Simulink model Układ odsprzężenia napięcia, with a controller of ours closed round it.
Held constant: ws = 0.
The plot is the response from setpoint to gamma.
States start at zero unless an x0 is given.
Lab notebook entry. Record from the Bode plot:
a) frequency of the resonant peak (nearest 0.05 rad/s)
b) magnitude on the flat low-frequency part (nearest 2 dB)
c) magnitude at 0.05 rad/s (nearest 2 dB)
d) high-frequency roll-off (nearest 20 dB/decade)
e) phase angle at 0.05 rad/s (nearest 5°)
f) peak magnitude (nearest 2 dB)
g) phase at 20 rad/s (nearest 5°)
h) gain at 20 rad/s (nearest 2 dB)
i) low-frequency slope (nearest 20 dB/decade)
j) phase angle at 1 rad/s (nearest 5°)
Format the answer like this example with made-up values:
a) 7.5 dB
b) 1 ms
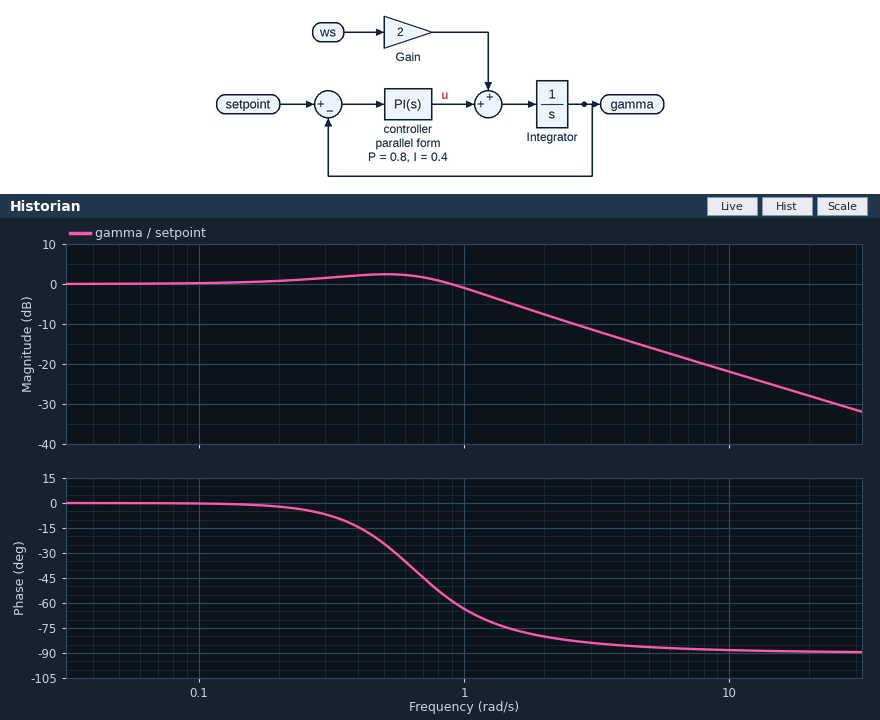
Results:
a) 0.50 rad/s
b) 0 dB
c) 0 dB
d) -20 dB/decade
e) 0°
f) 2 dB
g) -90°
h) -28 dB
i) 0 dB/decade
j) -65°
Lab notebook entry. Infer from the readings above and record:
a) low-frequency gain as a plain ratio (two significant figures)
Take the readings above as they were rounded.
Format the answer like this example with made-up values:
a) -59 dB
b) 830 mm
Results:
a) 1.0
